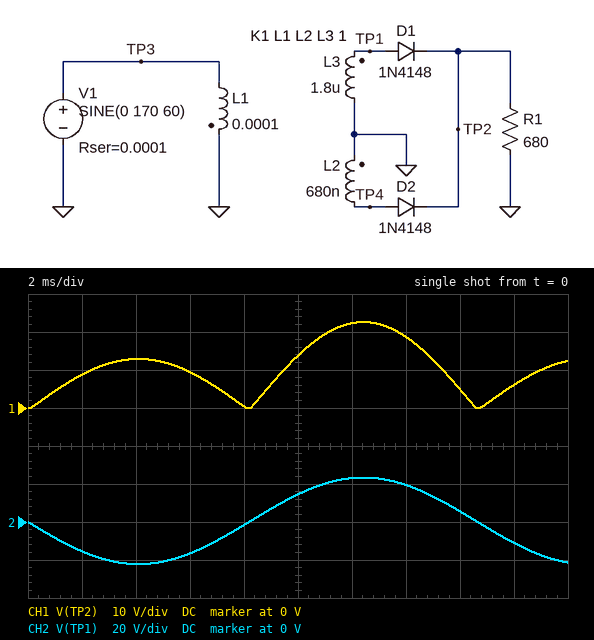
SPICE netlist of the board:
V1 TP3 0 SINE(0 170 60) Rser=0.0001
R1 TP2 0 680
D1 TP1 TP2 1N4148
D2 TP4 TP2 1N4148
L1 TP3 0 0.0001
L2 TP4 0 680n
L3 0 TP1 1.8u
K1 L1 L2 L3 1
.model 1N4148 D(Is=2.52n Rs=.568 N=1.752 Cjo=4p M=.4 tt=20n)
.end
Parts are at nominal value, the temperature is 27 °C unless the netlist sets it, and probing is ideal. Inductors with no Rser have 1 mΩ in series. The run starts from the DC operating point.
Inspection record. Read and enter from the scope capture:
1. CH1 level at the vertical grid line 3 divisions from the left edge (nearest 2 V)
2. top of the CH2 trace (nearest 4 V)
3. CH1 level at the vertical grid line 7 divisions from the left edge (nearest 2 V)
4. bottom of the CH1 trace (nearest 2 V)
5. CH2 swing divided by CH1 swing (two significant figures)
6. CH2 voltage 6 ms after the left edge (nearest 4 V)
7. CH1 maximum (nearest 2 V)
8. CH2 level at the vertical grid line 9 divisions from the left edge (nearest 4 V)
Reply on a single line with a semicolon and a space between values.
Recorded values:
10 V; 24 V; 18 V; 0 V; 2.0; -16 V; 22 V; -12 V
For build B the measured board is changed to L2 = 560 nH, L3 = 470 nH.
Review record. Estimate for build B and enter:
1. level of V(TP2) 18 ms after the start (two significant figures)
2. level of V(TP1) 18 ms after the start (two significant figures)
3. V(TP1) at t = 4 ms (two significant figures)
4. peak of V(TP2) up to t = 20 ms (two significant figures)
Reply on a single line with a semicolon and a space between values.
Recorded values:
5.5 V; -5.6 V; -11 V; 12 V
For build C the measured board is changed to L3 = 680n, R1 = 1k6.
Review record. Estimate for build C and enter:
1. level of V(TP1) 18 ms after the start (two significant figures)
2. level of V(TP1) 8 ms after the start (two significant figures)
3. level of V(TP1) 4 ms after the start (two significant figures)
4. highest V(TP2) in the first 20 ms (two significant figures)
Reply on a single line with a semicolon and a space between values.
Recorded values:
-6.8 V; -980 mV; -14 V; 14 V
